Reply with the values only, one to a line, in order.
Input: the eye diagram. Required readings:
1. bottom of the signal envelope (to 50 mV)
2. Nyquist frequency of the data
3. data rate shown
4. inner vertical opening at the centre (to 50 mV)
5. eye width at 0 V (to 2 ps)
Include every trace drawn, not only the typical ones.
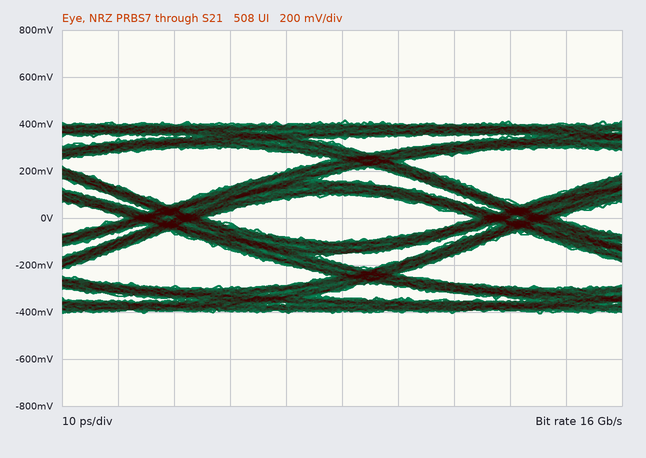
-400 mV
8 GHz
16 Gb/s
200 mV
48 ps
